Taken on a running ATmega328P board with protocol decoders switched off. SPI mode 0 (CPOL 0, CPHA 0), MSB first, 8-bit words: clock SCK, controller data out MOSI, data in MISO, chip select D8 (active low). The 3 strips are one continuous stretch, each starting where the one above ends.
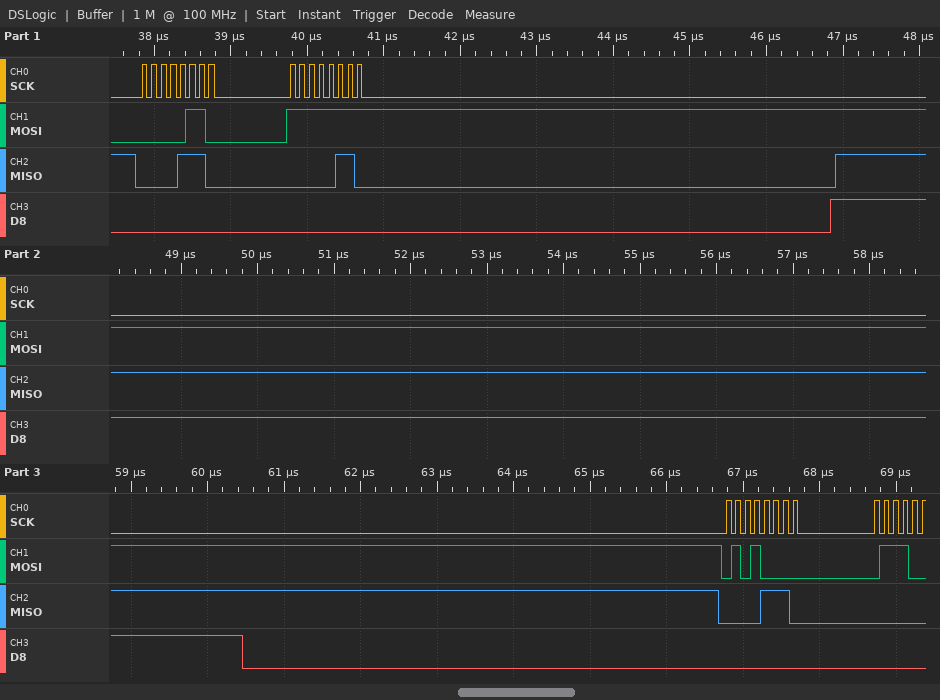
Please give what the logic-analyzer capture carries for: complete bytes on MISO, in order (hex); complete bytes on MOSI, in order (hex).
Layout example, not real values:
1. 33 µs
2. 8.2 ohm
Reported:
1. 0E 06 0E
2. 06 FF 50
